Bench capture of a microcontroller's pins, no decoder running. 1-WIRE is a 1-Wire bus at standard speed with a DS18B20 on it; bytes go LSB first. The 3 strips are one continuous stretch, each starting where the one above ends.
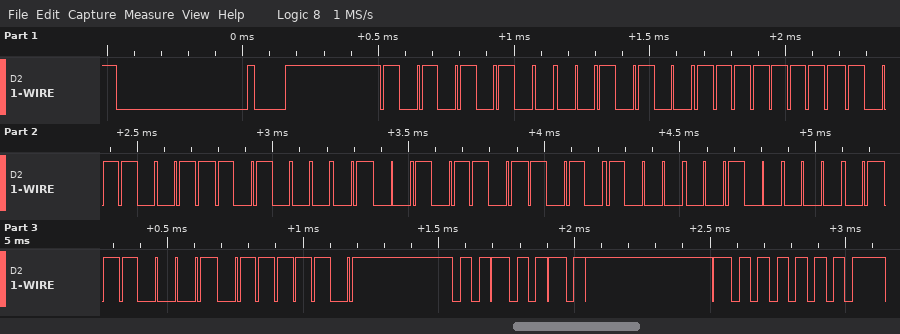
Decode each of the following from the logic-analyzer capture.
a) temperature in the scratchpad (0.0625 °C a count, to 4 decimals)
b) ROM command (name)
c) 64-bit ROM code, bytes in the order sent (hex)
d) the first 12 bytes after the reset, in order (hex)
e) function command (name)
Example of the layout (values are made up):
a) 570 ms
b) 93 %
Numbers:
a) 26.2500 °C
b) Match ROM
c) 28 FF CD 85 B4 15 04 8E
d) 55 28 FF CD 85 B4 15 04 8E BE A4 01
e) Read Scratchpad
